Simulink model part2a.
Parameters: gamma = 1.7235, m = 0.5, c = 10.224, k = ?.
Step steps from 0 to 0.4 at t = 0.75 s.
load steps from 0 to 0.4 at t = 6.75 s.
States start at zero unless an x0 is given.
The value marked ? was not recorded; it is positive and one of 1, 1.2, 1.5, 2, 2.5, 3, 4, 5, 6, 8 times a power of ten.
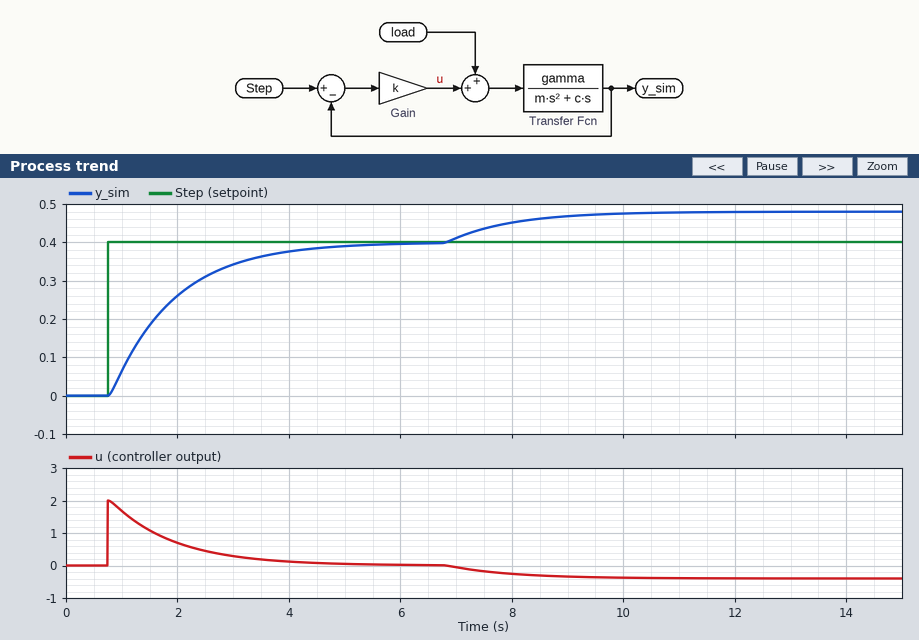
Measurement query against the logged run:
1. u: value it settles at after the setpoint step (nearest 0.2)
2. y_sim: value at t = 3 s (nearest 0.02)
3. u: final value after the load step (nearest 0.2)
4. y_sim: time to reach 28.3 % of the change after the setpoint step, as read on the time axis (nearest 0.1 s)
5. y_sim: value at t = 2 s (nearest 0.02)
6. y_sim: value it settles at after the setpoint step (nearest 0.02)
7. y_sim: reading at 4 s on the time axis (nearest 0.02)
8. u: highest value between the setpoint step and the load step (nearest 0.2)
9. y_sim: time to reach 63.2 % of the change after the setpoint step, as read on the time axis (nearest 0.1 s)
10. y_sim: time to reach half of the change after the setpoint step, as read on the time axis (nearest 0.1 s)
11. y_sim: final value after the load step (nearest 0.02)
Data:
0.0
0.34
-0.4
1.2 s
0.26
0.40
0.38
2.0
1.9 s
1.6 s
0.48
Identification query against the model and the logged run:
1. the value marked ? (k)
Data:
5
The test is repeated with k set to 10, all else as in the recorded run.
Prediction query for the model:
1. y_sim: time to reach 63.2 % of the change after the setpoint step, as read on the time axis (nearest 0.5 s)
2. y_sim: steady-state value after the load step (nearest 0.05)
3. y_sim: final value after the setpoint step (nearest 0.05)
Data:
1.5 s
0.45
0.40
